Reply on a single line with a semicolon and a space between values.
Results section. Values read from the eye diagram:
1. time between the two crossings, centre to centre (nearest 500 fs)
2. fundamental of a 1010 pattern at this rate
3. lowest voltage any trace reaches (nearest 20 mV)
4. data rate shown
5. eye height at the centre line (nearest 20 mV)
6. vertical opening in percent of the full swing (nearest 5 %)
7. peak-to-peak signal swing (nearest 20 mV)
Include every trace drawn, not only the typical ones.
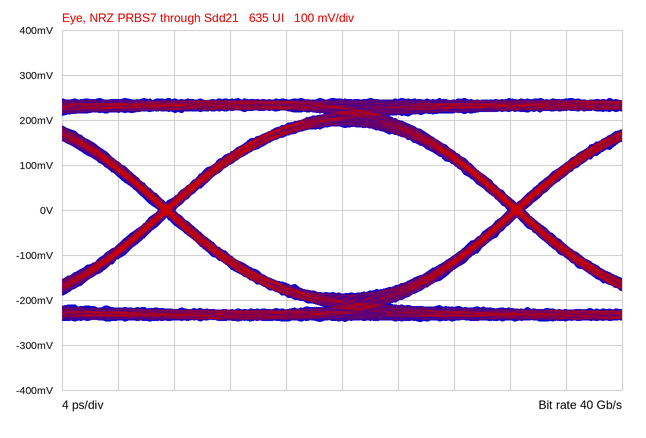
25.0 ps; 20 GHz; -240 mV; 40 Gb/s; 380 mV; 75 %; 500 mV
